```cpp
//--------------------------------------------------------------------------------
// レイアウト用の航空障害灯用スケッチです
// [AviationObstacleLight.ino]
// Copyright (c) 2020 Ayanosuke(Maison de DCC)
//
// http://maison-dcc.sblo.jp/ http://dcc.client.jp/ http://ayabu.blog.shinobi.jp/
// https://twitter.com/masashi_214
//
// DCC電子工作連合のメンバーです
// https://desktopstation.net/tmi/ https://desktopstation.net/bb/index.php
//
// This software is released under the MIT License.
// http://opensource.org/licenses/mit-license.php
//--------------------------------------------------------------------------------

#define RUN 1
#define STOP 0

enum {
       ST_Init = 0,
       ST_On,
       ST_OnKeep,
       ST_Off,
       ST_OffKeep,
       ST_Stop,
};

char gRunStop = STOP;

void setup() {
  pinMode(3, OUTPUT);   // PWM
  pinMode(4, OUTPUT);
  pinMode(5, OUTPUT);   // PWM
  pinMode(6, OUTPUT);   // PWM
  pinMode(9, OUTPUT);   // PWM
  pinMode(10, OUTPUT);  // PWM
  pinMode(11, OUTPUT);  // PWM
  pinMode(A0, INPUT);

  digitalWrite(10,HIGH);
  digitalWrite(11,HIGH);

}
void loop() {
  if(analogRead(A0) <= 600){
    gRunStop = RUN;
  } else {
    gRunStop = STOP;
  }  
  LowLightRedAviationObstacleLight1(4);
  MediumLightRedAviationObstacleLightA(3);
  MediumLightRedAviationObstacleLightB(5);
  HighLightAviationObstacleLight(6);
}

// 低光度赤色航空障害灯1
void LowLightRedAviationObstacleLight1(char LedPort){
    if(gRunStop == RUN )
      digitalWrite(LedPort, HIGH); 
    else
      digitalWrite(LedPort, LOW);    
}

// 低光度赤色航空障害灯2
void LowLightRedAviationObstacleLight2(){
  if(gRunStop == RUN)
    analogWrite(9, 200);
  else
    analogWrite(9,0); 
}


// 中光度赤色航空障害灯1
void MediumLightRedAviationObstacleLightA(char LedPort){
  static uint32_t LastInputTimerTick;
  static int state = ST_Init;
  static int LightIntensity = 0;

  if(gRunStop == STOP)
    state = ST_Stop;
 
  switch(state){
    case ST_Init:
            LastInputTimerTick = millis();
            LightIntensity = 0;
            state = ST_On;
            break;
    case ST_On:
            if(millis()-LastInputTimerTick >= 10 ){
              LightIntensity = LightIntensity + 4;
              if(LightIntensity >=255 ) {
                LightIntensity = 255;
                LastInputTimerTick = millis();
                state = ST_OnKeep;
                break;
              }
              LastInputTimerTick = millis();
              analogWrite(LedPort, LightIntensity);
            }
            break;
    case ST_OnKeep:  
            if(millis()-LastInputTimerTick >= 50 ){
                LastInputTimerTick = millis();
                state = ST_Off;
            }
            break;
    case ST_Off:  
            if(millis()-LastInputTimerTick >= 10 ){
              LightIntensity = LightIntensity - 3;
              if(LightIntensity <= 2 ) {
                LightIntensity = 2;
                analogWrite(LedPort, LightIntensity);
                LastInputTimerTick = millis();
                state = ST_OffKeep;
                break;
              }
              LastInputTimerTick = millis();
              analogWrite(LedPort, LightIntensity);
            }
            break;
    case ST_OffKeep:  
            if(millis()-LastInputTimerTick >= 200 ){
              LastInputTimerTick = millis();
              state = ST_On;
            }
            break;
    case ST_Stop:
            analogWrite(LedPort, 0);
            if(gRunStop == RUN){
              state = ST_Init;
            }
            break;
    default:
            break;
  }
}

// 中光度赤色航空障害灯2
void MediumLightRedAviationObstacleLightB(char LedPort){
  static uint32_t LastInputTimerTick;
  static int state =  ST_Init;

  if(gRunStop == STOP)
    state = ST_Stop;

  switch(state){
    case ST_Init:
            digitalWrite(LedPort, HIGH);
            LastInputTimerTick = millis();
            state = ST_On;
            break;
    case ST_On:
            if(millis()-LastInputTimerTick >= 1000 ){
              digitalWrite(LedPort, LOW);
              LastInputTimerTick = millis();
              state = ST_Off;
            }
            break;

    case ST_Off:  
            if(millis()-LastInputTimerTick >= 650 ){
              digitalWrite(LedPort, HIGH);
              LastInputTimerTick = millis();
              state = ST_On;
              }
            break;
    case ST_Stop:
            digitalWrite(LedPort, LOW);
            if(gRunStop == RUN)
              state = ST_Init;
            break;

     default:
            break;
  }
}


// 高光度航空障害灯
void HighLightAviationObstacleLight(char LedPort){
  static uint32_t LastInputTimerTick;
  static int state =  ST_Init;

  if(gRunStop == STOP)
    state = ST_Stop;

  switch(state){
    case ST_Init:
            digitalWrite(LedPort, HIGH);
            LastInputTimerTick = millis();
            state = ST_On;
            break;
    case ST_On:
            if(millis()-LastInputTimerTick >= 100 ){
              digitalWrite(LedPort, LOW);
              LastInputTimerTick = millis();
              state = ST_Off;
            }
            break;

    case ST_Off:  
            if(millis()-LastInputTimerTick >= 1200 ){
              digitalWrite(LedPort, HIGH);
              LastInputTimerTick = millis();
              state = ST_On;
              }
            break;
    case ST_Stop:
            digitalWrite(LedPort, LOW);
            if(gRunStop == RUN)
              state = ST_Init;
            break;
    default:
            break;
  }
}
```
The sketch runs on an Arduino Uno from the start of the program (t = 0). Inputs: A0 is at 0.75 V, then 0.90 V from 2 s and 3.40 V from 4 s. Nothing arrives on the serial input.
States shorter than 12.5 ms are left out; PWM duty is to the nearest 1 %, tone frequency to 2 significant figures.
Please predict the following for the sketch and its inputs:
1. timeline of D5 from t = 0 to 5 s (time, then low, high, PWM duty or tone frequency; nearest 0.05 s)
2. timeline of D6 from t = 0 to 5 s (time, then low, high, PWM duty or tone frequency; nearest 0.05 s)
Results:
0 s high; 1 s low; 1.65 s high; 2.65 s low; 3.3 s high; 4 s low
0 s high; 0.1 s low; 1.3 s high; 1.4 s low; 2.6 s high; 2.7 s low; 3.9 s high; 4 s low
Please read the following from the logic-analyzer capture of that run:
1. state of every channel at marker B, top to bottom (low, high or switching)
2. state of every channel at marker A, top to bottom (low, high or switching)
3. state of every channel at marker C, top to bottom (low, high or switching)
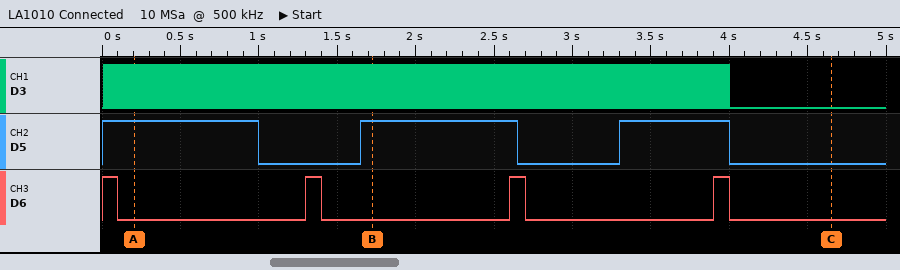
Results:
D3 switching, D5 high, D6 low
D3 switching, D5 high, D6 low
D3 low, D5 low, D6 low
